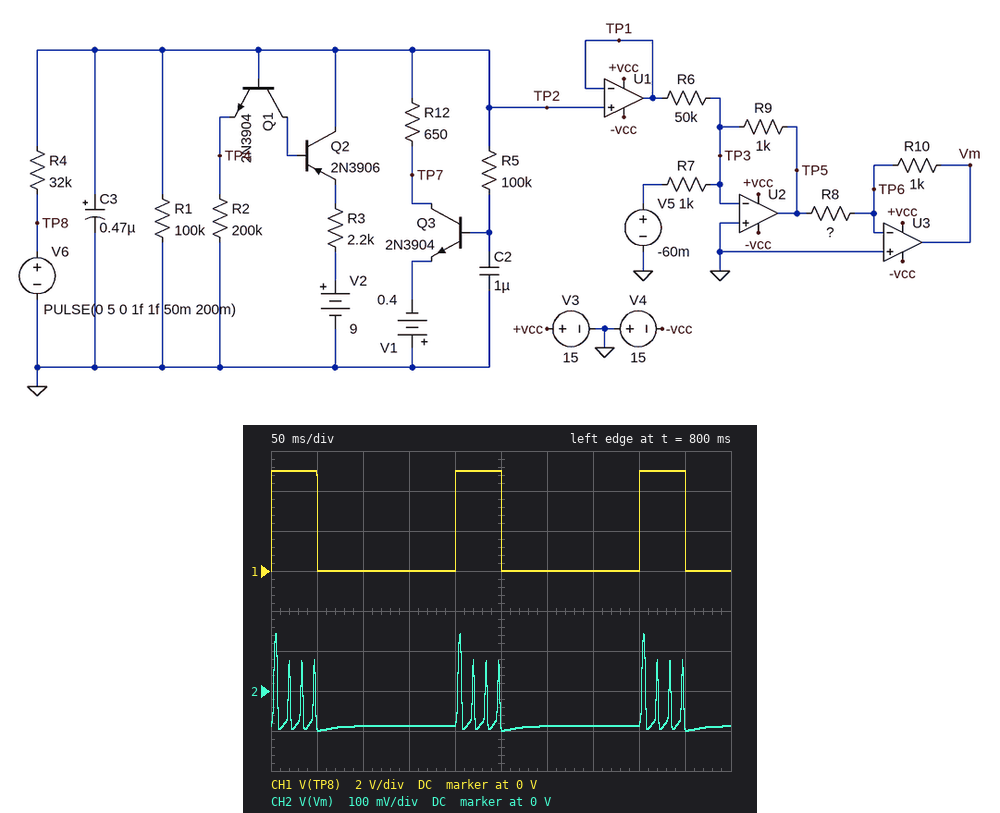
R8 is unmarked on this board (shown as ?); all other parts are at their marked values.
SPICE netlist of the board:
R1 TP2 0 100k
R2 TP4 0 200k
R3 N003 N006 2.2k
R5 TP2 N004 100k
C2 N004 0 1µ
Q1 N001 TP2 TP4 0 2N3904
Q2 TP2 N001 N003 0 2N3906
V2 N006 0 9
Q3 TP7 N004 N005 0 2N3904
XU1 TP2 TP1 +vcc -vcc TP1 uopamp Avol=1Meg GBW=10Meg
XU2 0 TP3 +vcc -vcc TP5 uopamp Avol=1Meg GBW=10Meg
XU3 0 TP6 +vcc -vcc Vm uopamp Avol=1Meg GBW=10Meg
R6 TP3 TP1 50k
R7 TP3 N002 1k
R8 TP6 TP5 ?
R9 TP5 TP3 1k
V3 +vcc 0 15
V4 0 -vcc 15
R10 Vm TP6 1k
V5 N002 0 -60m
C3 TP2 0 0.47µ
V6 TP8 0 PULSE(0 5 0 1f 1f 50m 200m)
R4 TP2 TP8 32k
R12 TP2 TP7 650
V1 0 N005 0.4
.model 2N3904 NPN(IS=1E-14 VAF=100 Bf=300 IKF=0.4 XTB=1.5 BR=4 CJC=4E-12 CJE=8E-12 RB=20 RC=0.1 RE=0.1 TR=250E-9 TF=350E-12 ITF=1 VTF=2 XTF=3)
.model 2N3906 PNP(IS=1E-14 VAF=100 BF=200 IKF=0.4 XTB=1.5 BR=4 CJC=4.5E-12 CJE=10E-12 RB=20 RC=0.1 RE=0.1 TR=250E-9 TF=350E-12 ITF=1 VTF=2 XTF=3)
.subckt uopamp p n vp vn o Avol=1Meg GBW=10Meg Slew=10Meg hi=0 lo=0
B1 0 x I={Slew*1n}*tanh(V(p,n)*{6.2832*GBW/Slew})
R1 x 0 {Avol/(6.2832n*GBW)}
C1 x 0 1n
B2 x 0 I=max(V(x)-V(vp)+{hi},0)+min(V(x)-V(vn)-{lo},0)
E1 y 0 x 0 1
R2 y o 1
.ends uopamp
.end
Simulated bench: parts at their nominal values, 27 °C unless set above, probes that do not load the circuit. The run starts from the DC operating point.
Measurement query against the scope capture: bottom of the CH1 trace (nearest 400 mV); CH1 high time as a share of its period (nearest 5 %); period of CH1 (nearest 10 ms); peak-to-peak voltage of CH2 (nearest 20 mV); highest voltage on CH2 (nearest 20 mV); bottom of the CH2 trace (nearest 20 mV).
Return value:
0 V
25 %
200 ms
240 mV
140 mV
-100 mV
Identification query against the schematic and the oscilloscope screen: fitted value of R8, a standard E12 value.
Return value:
680 Ω
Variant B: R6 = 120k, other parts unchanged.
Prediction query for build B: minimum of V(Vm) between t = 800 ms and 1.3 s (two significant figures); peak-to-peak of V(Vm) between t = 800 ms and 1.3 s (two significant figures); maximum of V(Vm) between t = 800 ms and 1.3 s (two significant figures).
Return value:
-93 mV
100 mV
7.9 mV
